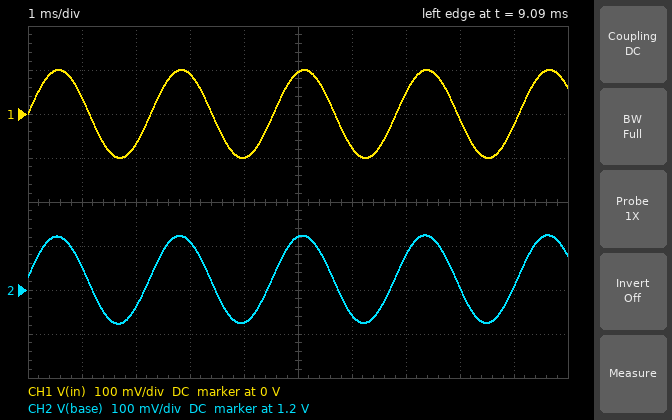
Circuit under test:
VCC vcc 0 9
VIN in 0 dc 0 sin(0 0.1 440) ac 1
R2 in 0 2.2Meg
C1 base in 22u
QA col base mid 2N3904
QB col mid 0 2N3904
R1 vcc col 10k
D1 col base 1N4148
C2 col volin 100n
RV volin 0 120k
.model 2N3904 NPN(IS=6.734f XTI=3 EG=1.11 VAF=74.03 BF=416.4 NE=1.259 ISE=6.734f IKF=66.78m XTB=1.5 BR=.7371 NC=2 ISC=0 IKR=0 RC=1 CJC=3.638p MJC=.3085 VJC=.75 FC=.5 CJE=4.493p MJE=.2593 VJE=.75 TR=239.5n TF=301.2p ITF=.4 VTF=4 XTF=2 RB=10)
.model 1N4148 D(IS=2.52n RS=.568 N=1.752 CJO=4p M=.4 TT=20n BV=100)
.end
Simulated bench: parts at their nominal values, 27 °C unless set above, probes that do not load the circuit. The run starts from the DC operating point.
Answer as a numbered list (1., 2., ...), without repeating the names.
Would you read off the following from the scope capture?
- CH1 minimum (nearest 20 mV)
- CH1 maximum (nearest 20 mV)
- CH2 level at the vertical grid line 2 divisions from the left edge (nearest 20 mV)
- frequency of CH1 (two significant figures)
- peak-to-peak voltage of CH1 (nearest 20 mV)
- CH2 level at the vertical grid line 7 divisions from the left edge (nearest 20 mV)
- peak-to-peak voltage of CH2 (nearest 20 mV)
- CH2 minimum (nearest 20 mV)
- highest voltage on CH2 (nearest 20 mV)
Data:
1. -100 mV
2. 100 mV
3. 1.16 V
4. 440 Hz
5. 200 mV
6. 1.28 V
7. 200 mV
8. 1.12 V
9. 1.32 V
